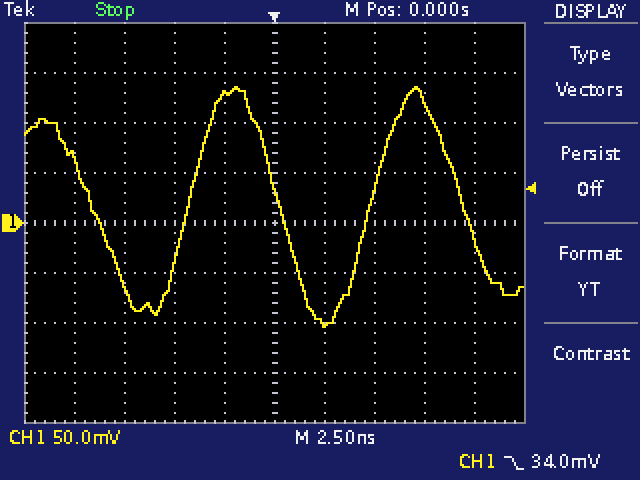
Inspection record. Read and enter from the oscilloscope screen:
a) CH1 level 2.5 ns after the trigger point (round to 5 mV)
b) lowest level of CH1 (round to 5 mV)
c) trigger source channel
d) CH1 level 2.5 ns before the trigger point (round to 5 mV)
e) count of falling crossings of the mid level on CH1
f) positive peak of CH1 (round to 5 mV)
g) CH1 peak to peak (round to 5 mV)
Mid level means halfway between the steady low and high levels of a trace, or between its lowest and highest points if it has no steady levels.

-100 mV
-105 mV
CH1
130 mV
3
135 mV
240 mV
